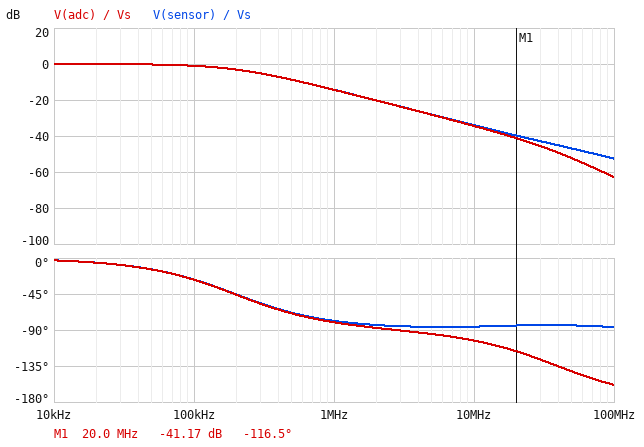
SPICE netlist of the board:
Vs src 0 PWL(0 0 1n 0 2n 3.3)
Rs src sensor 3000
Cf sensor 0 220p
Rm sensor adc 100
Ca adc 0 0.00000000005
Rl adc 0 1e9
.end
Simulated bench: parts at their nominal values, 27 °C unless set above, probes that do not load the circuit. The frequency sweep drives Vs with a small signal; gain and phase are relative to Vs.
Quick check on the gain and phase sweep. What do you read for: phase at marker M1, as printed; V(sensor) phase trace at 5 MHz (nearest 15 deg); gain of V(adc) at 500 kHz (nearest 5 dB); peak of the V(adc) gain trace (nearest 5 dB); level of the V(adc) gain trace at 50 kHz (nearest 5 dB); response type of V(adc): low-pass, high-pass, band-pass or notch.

-116.5 deg
-90 deg
-10 dB
0 dB
0 dB
low-pass
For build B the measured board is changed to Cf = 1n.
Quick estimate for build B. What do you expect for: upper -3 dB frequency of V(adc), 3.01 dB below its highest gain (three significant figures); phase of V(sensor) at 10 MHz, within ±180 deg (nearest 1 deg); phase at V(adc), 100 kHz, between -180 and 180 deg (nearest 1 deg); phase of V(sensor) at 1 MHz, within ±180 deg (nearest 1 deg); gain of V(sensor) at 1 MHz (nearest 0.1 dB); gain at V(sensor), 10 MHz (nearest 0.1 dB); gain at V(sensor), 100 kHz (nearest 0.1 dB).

50.5 kHz
-89 deg
-63 deg
-87 deg
-25.9 dB
-45.9 dB
-6.9 dB
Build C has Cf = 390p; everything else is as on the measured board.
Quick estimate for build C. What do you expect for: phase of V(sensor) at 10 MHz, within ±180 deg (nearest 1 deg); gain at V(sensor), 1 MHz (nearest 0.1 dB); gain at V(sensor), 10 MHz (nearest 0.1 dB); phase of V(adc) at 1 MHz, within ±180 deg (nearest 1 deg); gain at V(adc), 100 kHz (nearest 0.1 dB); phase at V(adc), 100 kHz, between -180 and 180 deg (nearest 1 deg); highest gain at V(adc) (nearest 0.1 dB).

-87 deg
-18.4 dB
-38.3 dB
-85 deg
-2.3 dB
-40 deg
0 dB
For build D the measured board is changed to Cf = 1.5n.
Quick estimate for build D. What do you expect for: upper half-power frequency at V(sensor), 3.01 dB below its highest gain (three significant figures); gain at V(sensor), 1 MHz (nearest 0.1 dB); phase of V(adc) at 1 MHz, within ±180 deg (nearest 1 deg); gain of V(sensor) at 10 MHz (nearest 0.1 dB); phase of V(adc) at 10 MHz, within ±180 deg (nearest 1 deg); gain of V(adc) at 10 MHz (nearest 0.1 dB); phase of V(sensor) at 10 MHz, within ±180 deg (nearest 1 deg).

34.2 kHz
-29.3 dB
-90 deg
-49.3 dB
-107 deg
-49.7 dB
-89 deg
